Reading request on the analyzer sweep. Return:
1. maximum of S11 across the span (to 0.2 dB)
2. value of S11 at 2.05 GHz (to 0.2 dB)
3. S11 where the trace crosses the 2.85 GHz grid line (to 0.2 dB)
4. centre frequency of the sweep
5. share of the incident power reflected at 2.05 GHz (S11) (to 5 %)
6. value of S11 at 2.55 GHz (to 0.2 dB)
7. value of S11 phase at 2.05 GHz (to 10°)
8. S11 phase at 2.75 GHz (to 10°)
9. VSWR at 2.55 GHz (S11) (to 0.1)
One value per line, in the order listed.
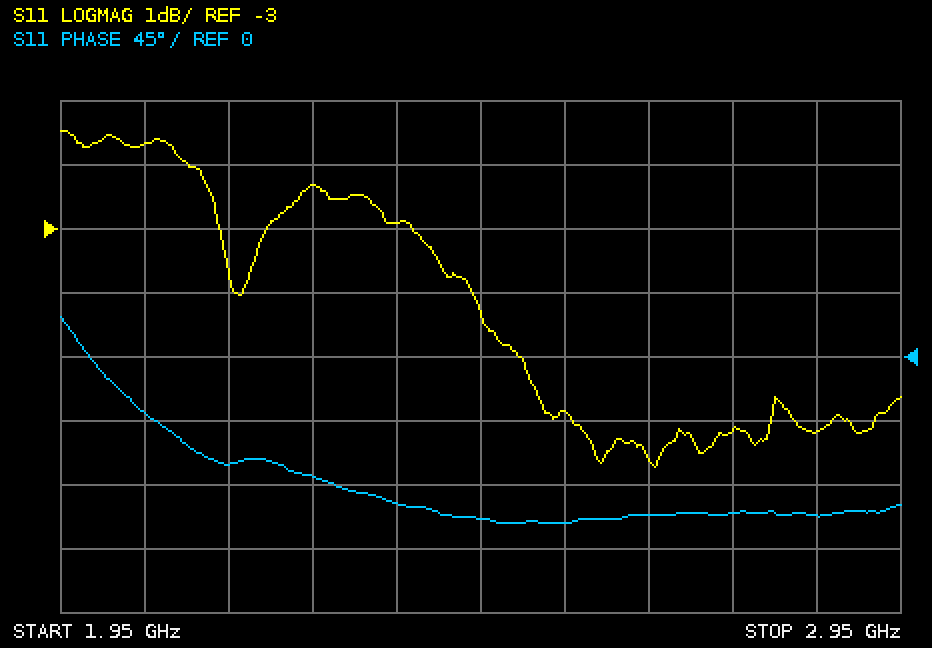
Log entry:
-1.4 dB
-1.6 dB
-6.2 dB
2.45 GHz
70 %
-5.8 dB
-40°
-110°
3.1
